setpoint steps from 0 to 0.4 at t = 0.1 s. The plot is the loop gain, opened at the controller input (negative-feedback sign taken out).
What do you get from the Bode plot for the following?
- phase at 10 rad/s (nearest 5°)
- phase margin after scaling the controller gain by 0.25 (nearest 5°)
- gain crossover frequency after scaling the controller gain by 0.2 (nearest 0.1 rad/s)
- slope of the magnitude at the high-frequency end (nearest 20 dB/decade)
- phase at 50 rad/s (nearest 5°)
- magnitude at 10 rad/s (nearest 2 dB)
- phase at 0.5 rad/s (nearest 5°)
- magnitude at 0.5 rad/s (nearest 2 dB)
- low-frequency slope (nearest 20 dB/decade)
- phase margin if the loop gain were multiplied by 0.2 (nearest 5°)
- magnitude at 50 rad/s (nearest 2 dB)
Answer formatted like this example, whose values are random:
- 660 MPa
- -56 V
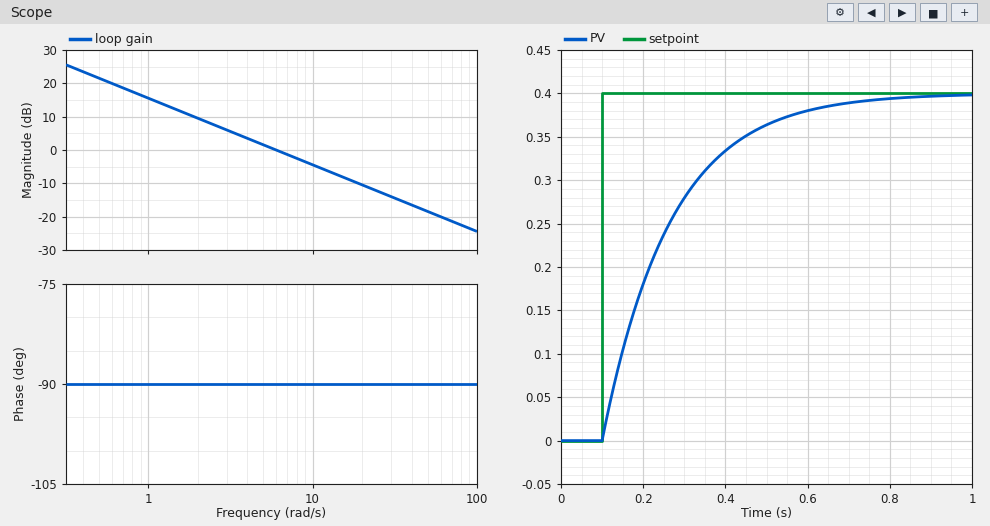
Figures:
- -90°
- 90°
- 1.2 rad/s
- -20 dB/decade
- -90°
- -4 dB
- -90°
- 22 dB
- -20 dB/decade
- 90°
- -18 dB
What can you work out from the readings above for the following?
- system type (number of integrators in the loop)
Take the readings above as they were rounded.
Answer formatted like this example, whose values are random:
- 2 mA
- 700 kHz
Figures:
- 1
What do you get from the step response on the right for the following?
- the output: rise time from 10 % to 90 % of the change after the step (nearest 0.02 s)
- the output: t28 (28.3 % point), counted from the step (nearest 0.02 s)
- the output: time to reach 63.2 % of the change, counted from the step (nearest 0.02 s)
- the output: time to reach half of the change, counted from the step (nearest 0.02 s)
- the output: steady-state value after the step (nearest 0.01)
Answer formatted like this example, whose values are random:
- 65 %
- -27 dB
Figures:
- 0.36 s
- 0.06 s
- 0.16 s
- 0.12 s
- 0.40
